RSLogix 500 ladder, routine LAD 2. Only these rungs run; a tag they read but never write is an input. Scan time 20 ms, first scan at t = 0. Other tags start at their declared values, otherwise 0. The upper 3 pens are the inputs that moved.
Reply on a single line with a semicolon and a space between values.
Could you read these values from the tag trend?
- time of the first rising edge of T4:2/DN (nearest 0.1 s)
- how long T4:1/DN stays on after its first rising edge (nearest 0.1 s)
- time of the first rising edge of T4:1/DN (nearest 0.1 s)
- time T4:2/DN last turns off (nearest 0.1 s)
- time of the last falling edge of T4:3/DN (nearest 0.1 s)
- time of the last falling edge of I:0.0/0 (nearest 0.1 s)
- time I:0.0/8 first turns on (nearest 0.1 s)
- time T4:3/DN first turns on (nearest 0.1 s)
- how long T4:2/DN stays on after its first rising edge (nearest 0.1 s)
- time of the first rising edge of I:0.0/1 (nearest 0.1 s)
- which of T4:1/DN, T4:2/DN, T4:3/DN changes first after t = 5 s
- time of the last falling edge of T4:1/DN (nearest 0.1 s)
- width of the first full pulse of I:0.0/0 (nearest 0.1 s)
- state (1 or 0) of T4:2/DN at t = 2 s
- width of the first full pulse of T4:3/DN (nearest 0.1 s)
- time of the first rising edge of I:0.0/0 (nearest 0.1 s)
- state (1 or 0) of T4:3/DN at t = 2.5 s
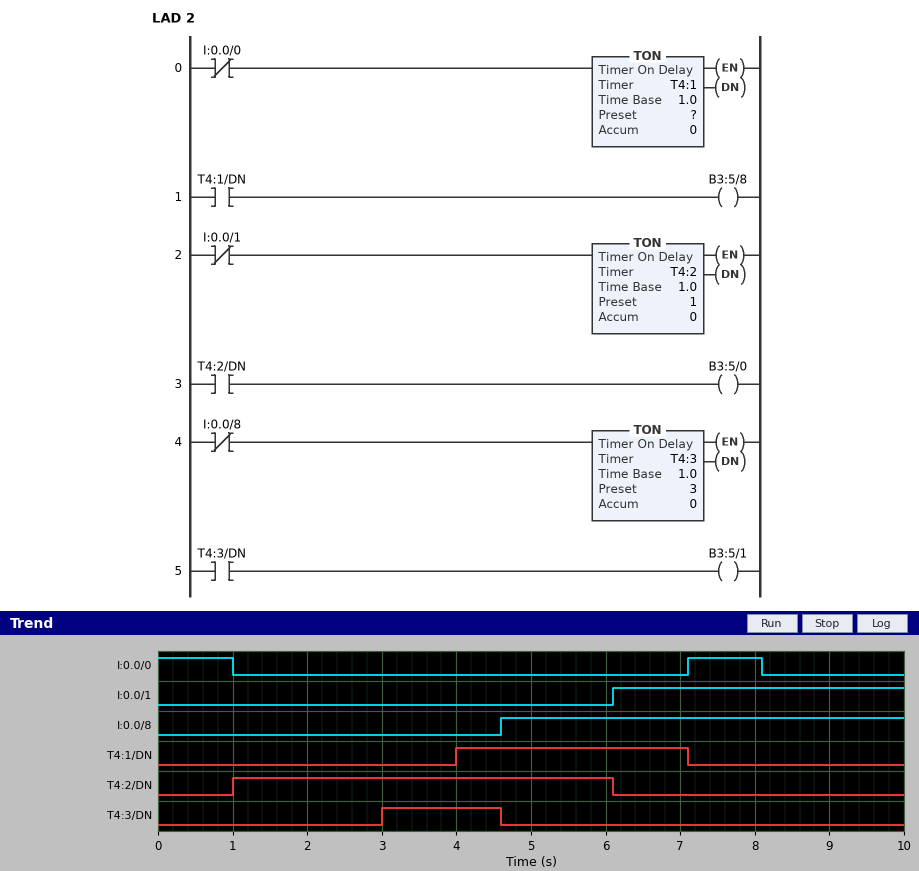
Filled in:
1.0 s; 3.1 s; 4.0 s; 6.1 s; 4.6 s; 8.1 s; 4.6 s; 3.0 s; 5.1 s; 6.1 s; T4:2/DN; 7.1 s; 1.0 s; 1; 1.6 s; 7.1 s; 0
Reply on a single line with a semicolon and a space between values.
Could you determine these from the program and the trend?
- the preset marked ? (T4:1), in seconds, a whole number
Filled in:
3 s
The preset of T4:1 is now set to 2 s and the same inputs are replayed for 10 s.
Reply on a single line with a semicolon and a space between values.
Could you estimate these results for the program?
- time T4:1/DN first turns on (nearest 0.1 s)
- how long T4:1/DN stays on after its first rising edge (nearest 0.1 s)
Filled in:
3.0 s; 4.1 s
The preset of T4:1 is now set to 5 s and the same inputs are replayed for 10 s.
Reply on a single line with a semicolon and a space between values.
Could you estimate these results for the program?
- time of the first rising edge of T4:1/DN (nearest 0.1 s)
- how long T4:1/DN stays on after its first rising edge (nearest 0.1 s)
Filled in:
6.0 s; 1.1 s
